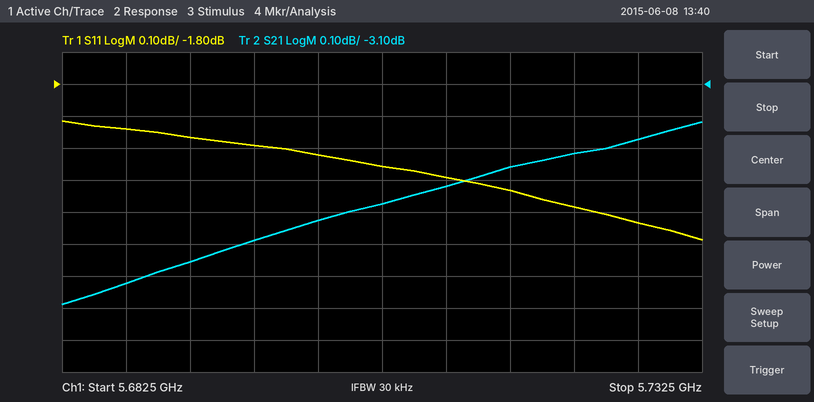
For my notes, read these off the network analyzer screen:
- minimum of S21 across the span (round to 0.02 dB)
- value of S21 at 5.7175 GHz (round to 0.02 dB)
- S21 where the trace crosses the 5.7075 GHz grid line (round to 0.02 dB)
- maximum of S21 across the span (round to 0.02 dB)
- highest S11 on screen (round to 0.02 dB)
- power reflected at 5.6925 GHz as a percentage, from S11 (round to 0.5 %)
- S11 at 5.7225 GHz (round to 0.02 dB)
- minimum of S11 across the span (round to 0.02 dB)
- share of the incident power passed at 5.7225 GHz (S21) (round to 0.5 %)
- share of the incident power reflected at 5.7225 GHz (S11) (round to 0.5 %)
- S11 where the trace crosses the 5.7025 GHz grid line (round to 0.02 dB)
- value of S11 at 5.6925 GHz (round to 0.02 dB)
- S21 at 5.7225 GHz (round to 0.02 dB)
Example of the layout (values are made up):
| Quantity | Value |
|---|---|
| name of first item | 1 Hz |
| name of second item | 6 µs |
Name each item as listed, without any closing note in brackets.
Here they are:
| Quantity | Value |
|---|---|
| minimum of S21 across the span | -3.78 dB |
| value of S21 at 5.7175 GHz | -3.36 dB |
| S21 where the trace crosses the 5.7075 GHz grid line | -3.48 dB |
| maximum of S21 across the span | -3.22 dB |
| highest S11 on screen | -1.92 dB |
| power reflected at 5.6925 GHz as a percentage, from S11 | 63.5 % |
| S11 at 5.7225 GHz | -2.18 dB |
| minimum of S11 across the span | -2.28 dB |
| share of the incident power passed at 5.7225 GHz (S21) | 46.5 % |
| share of the incident power reflected at 5.7225 GHz (S11) | 60.5 % |
| S11 where the trace crosses the 5.7025 GHz grid line | -2.02 dB |
| value of S11 at 5.6925 GHz | -1.96 dB |
| S21 at 5.7225 GHz | -3.32 dB |
